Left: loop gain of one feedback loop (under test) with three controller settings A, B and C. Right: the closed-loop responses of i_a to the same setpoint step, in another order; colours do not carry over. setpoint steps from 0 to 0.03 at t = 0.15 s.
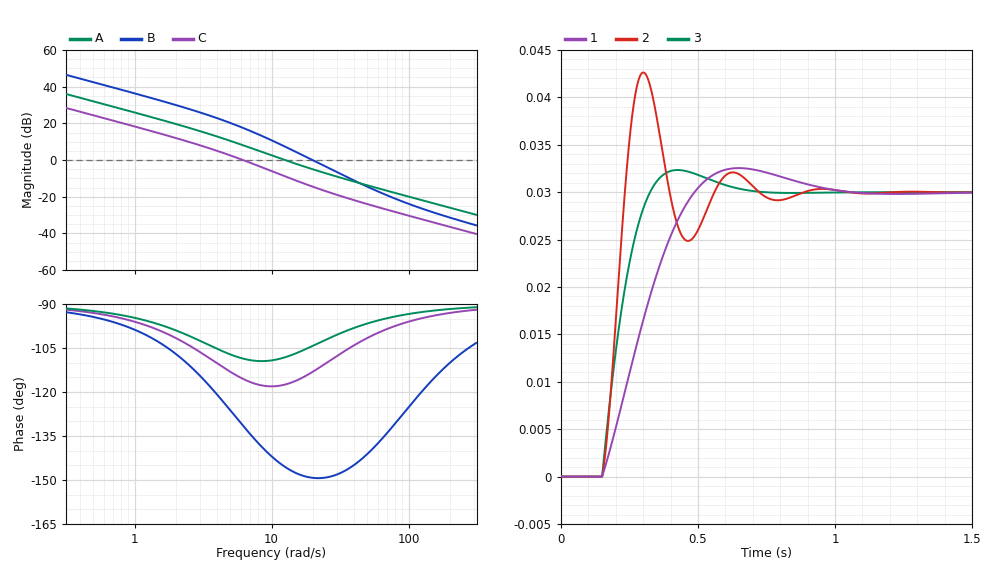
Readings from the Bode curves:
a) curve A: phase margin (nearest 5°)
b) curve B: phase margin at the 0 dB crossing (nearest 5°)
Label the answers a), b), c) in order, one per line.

a) 70°
b) 30°
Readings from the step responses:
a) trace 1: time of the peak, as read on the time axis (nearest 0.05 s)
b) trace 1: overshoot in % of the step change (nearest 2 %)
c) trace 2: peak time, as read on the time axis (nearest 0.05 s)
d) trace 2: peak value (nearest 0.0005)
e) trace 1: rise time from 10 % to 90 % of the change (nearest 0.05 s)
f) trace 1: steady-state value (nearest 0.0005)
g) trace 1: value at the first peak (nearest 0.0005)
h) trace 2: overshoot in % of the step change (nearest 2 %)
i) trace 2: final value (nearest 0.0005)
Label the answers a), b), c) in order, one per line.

a) 0.65 s
b) 8 %
c) 0.30 s
d) 0.0425
e) 0.25 s
f) 0.0300
g) 0.0325
h) 42 %
i) 0.0300
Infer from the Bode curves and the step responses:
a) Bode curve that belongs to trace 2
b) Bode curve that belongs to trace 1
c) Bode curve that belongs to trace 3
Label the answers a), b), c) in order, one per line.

a) B
b) C
c) A
